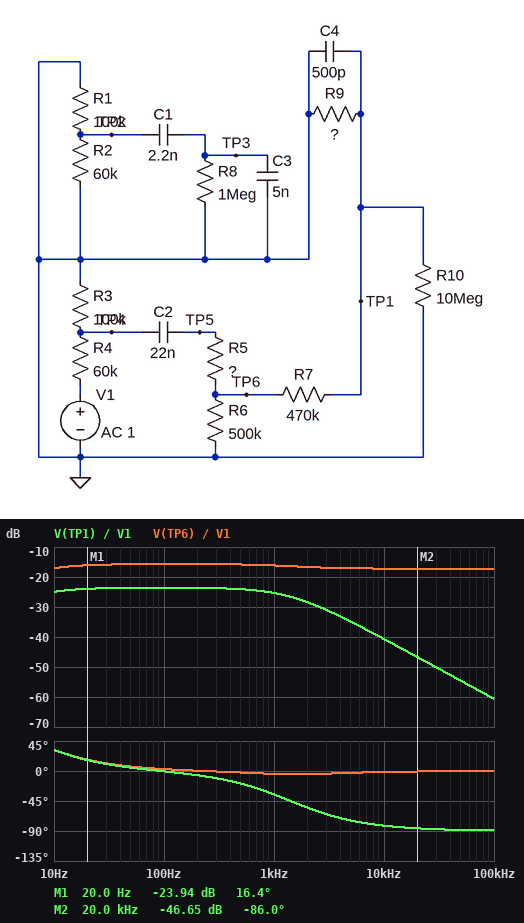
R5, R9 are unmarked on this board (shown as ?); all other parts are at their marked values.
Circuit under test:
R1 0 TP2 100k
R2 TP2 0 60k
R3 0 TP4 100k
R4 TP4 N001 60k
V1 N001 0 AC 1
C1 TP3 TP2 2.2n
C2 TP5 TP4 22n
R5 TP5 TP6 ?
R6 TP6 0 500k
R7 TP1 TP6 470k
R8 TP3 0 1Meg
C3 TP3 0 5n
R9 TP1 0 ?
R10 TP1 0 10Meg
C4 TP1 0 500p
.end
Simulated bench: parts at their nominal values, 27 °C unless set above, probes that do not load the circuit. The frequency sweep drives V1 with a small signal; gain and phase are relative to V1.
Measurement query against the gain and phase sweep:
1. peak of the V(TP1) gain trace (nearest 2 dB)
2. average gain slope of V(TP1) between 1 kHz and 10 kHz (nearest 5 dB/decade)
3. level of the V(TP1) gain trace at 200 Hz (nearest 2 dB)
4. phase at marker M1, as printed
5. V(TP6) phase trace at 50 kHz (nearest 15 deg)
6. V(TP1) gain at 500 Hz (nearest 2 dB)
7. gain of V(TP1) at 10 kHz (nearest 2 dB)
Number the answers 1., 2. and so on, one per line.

1. -24 dB
2. -15 dB/decade
3. -24 dB
4. 16.4 deg
5. 0 deg
6. -24 dB
7. -40 dB
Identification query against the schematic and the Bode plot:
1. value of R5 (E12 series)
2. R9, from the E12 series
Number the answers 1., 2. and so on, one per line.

1. 820 kΩ
2. 330 kΩ
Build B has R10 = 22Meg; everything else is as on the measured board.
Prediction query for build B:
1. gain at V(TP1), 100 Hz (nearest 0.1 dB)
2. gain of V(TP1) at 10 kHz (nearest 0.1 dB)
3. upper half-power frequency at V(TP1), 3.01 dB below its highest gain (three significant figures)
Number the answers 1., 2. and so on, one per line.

1. -23.5 dB
2. -40.7 dB
3. 1.40 kHz
